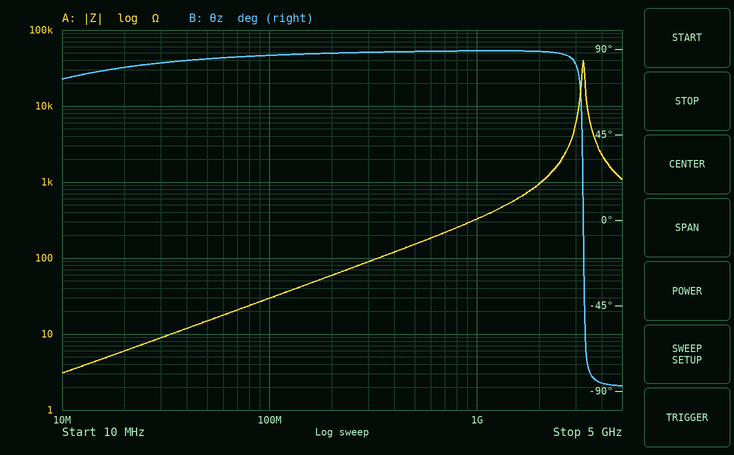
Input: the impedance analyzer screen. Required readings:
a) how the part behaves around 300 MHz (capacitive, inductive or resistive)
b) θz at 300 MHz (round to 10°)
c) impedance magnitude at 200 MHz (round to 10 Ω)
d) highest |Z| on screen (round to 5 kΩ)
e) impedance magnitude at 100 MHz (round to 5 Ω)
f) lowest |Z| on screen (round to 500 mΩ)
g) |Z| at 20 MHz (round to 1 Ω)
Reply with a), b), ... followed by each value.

a) inductive
b) 90°
c) 60 Ω
d) 40 kΩ
e) 30 Ω
f) 3.0 Ω
g) 6 Ω
